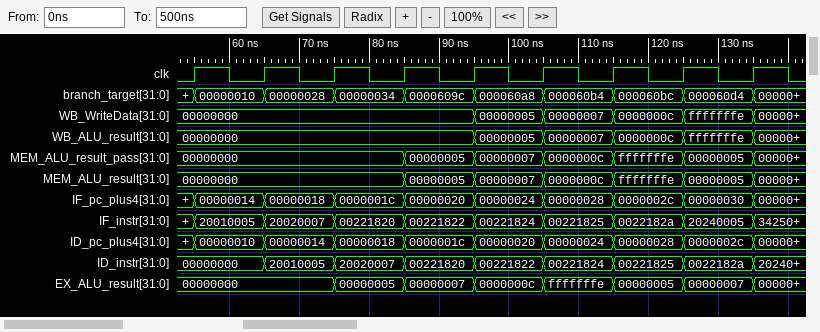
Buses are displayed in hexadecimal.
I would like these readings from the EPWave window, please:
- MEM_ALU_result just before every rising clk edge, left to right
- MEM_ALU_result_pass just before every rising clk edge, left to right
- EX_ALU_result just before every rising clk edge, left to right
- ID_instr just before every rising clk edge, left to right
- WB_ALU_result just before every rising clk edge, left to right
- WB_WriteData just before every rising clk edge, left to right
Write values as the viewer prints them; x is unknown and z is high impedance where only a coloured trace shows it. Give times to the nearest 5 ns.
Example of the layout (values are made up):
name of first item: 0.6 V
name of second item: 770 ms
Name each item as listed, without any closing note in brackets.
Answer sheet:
MEM_ALU_result just before every rising clk edge, left to right: 00000000, 00000000, 00000000, 00000000, 00000005, 00000007, 0000000c, fffffffe, 00000005
MEM_ALU_result_pass just before every rising clk edge, left to right: 00000000, 00000000, 00000000, 00000000, 00000005, 00000007, 0000000c, fffffffe, 00000005
EX_ALU_result just before every rising clk edge, left to right: 00000000, 00000000, 00000000, 00000005, 00000007, 0000000c, fffffffe, 00000005, 00000007
ID_instr just before every rising clk edge, left to right: 00000000, 00000000, 20010005, 20020007, 00221820, 00221822, 00221824, 00221825, 0022182a
WB_ALU_result just before every rising clk edge, left to right: 00000000, 00000000, 00000000, 00000000, 00000000, 00000005, 00000007, 0000000c, fffffffe
WB_WriteData just before every rising clk edge, left to right: 00000000, 00000000, 00000000, 00000000, 00000000, 00000005, 00000007, 0000000c, fffffffe
